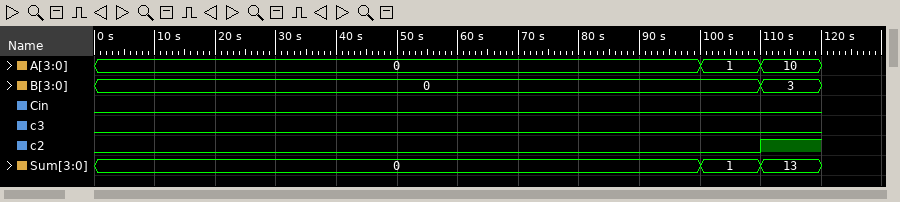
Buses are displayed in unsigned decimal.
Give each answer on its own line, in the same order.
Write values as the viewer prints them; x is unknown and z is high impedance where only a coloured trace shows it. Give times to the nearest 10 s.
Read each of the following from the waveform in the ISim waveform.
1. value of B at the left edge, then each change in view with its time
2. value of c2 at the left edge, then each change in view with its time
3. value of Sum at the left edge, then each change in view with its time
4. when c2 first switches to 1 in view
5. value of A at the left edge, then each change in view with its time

0, 3 at 110 s
0, 1 at 110 s
0, 1 at 100 s, 13 at 110 s
110 s
0, 1 at 100 s, 10 at 110 s
